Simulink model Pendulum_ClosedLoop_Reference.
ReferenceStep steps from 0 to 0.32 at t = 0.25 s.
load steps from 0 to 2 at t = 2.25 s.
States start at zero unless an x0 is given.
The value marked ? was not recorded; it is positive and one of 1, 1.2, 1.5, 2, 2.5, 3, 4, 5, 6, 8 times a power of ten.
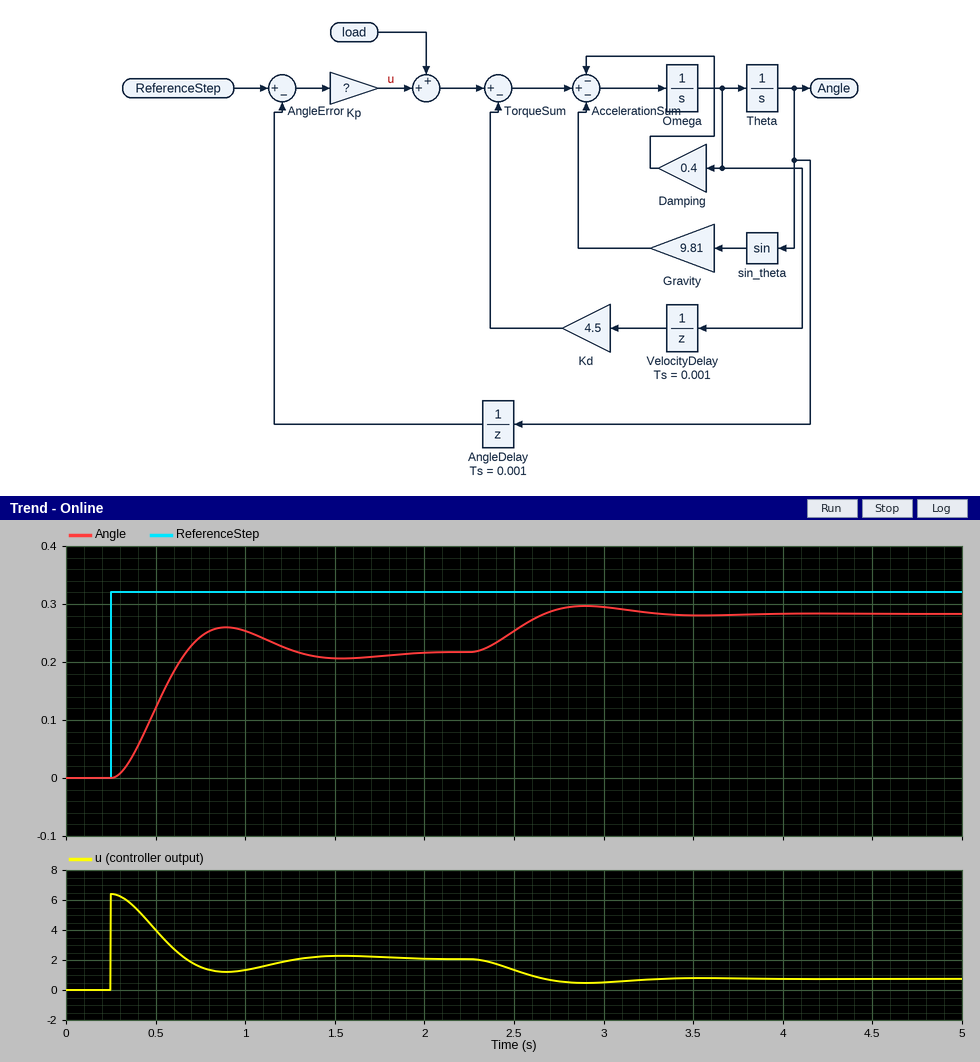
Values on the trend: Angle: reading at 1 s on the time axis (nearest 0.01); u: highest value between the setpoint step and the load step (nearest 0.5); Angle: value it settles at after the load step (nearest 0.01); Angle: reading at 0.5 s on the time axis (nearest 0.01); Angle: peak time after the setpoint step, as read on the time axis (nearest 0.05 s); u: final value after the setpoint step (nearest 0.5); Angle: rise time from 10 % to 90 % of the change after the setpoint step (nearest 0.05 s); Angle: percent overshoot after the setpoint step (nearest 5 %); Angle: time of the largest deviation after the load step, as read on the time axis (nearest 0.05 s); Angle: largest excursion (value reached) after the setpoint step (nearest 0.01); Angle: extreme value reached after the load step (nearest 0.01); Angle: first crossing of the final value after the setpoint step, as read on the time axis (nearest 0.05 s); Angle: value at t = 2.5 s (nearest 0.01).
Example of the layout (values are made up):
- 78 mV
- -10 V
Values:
- 0.25
- 6.5
- 0.28
- 0.12
- 0.90 s
- 2.0
- 0.30 s
- 20 %
- 2.90 s
- 0.26
- 0.30
- 0.65 s
- 0.25
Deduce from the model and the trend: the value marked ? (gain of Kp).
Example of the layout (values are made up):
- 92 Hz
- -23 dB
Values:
- 20
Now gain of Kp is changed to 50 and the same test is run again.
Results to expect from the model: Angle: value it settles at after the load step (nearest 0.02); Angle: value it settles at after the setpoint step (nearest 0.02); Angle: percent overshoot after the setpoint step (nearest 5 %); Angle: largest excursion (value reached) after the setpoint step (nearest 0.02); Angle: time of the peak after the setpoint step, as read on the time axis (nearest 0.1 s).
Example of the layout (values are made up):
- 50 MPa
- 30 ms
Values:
- 0.30
- 0.26
- 35 %
- 0.36
- 0.7 s
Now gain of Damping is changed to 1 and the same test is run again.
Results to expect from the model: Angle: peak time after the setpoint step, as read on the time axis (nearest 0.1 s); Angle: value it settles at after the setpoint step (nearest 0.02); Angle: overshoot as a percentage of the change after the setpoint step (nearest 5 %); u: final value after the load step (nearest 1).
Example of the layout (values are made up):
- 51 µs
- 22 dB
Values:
- 0.9 s
- 0.22
- 15 %
- 1
